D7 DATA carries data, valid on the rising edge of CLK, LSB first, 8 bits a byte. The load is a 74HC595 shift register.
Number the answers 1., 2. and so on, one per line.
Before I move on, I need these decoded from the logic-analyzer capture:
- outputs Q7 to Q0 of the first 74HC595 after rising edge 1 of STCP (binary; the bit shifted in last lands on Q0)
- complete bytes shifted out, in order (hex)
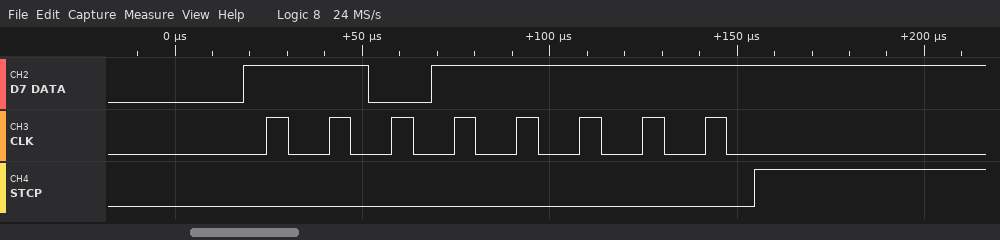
1. 11011111
2. FB
